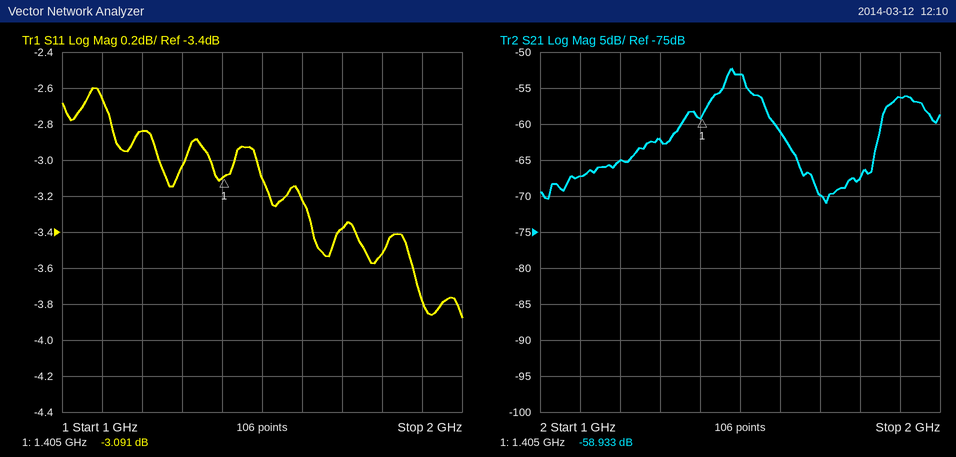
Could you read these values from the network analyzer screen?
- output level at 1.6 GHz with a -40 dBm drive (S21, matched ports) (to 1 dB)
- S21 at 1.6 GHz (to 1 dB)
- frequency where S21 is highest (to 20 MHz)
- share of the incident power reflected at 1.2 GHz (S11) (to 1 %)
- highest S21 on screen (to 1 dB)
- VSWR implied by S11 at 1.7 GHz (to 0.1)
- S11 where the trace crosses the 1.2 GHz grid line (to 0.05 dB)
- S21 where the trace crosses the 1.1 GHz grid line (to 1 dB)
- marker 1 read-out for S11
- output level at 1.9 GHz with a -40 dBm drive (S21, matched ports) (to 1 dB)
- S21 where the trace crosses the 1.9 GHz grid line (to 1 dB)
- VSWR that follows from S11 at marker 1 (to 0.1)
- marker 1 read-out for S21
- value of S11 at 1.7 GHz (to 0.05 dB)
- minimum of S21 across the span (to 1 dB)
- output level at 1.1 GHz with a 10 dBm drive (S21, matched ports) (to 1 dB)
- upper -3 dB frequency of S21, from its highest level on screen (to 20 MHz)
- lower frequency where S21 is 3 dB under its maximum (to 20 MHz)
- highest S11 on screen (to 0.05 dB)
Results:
-101 dBm
-61 dB
1.48 GHz
52 %
-52 dB
5.2
-2.85 dB
-67 dB
-3.091 dB
-96 dBm
-56 dB
5.7
-58.933 dB
-3.40 dB
-71 dB
-57 dBm
1.52 GHz
1.46 GHz
-2.60 dB
